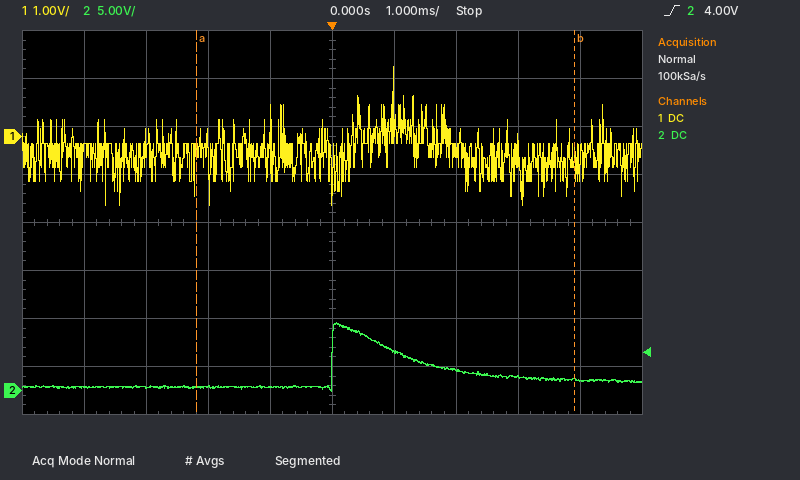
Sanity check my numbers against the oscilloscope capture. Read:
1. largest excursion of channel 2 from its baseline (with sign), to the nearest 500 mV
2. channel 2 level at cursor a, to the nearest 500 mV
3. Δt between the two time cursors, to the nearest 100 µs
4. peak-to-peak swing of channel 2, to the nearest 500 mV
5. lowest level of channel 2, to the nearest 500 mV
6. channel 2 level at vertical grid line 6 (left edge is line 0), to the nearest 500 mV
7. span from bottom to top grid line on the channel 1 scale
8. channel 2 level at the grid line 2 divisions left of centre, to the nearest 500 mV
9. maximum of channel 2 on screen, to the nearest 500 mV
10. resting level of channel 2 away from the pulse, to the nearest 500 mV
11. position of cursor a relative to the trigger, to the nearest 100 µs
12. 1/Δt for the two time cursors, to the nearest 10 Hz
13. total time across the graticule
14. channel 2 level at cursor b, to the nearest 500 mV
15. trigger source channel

+6.5 V
500 mV
6.1 ms
7.0 V
0.0 V
4.0 V
8 V
500 mV
7.0 V
500 mV
-2.2 ms
160 Hz
10 ms
1.0 V
channel 2
